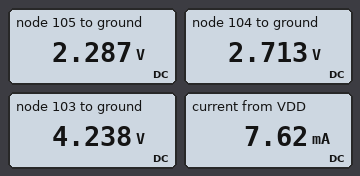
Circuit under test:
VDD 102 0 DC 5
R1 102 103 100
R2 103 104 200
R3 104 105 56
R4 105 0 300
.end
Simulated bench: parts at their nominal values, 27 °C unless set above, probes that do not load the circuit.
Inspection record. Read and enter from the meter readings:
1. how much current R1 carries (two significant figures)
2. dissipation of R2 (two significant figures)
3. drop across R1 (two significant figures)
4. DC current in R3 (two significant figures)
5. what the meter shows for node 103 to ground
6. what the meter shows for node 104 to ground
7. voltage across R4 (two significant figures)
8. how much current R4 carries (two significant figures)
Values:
7.6 mA
12 mW
760 mV
7.6 mA
4.238 V
2.713 V
2.3 V
7.6 mA
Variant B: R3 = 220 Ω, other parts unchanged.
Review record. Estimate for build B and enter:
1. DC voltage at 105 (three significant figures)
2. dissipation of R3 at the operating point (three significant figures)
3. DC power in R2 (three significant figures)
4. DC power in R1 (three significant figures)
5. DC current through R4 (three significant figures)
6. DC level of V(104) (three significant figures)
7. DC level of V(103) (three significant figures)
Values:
1.83 V
8.18 mW
7.44 mW
3.72 mW
6.10 mA
3.17 V
4.39 V
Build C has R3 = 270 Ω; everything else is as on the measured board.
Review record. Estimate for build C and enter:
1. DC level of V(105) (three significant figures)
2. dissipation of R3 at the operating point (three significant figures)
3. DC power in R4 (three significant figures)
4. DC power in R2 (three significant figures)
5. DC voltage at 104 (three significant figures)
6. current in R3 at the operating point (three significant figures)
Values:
1.72 V
8.92 mW
9.91 mW
6.61 mW
3.28 V
5.75 mA
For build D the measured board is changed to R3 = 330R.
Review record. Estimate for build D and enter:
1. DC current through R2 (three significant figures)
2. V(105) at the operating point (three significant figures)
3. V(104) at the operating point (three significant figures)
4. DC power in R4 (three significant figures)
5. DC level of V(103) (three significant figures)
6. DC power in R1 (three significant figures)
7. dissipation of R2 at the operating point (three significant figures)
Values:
5.38 mA
1.61 V
3.39 V
8.67 mW
4.46 V
2.89 mW
5.78 mW
